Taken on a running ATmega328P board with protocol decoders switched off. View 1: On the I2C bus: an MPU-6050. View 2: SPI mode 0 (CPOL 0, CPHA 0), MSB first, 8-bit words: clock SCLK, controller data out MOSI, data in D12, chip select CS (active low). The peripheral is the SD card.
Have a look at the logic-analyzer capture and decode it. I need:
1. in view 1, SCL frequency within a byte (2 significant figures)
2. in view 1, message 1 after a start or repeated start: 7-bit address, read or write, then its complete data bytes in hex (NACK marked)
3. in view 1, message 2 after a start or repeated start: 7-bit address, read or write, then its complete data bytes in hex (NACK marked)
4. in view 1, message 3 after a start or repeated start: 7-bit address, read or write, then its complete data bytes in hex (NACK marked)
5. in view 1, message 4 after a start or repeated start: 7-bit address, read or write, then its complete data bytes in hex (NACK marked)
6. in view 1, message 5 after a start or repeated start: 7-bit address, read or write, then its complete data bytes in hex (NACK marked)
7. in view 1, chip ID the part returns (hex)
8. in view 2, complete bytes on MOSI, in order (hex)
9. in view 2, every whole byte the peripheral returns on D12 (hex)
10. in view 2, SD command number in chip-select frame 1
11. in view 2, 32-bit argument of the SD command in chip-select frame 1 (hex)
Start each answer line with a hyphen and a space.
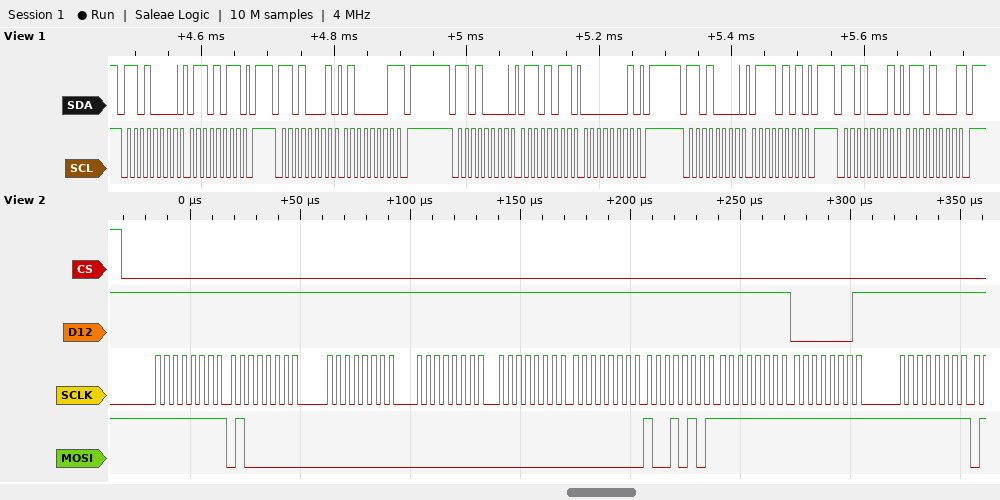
- 100 kHz
- 0x68 write: 6B
- 0x68 read: 41 NACK
- 0x68 write: 6B 01
- 0x68 write: 75
- 0x68 read: 68 NACK
- 0x68
- FF 40 00 00 00 00 95 FF FF FF
- FF FF FF FF FF FF FF FF 01 FF
- CMD0
- 0x00000000
